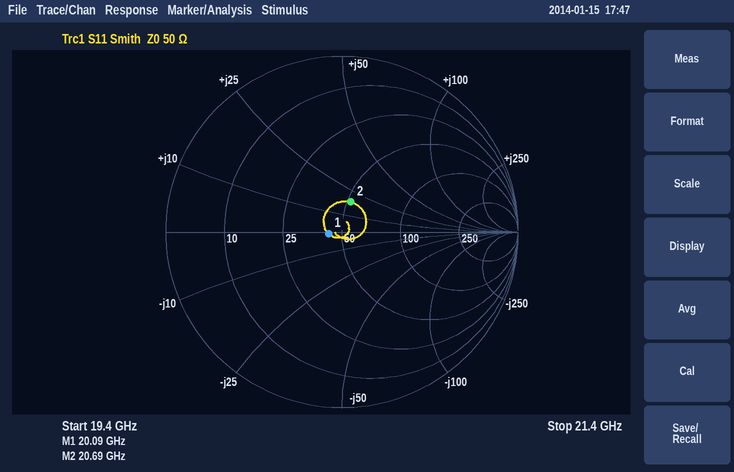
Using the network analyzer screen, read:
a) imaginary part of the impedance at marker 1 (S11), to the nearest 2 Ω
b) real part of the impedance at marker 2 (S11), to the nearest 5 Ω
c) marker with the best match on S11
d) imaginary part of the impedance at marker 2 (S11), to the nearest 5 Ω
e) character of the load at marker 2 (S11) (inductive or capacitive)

0 Ω
50 Ω
marker 1
+20 Ω
inductive
